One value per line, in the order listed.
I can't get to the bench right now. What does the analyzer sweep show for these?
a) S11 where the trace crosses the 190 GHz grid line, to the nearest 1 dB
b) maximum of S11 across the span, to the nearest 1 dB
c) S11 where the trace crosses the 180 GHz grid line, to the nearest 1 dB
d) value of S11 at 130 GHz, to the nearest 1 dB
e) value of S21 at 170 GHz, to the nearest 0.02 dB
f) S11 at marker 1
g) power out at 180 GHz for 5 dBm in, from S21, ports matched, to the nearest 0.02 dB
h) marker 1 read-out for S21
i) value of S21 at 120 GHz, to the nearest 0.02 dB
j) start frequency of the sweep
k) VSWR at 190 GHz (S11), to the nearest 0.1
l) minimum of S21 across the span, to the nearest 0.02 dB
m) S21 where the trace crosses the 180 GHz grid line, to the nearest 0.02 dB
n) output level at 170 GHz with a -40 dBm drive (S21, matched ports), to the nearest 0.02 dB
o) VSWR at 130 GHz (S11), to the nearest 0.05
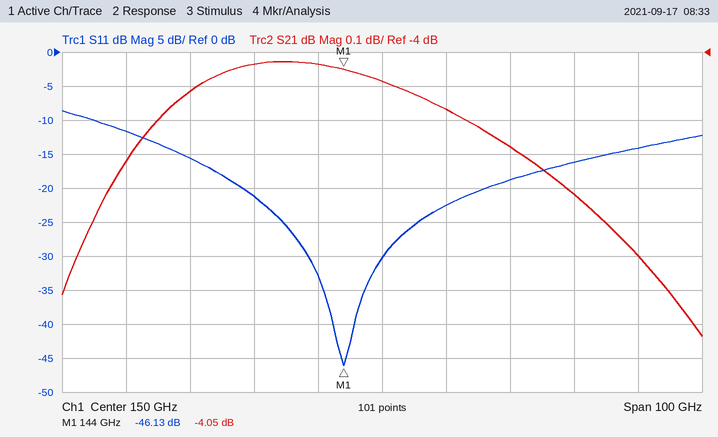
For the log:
-14 dB
-9 dB
-16 dB
-21 dB
-4.28 dB
-46.13 dB
0.58 dBm
-4.05 dB
-4.12 dB
100 GHz
1.5
-4.84 dB
-4.42 dB
-44.28 dBm
1.20
